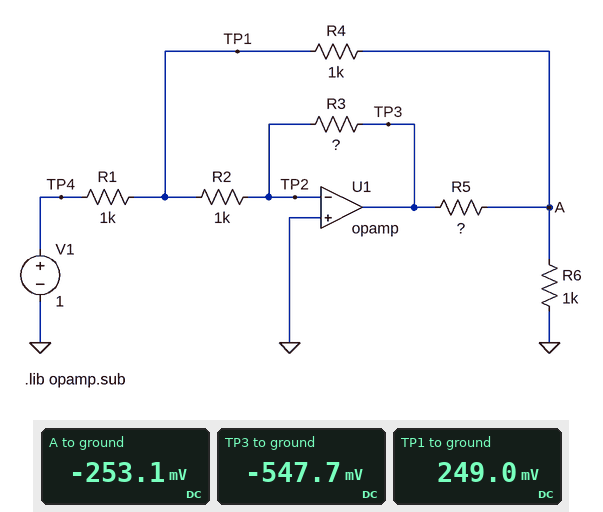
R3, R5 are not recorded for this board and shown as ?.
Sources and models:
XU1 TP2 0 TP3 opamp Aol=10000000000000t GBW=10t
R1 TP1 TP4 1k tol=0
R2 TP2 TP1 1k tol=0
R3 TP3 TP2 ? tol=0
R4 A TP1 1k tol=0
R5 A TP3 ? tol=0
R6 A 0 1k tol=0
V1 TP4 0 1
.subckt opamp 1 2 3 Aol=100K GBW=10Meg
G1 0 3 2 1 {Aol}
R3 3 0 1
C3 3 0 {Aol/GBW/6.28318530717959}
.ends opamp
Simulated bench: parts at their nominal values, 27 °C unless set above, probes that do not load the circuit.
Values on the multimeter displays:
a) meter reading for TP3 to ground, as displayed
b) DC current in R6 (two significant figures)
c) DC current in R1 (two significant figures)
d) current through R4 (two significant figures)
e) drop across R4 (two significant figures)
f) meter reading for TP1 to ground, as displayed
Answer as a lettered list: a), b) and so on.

a) -547.7 mV
b) 250 µA
c) 750 µA
d) 500 µA
e) 500 mV
f) 249.0 mV
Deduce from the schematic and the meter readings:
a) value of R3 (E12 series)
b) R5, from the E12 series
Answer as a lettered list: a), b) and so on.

a) 2.2 kΩ
b) 390 Ω
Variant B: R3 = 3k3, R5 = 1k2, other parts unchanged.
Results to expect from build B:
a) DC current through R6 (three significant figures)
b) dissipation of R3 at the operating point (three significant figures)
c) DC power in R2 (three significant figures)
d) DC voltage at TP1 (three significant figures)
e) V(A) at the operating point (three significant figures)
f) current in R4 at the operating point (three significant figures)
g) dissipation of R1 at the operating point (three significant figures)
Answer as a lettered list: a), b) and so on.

a) 171 µA
b) 252 µW
c) 76.4 µW
d) 276 mV
e) -171 mV
f) 447 µA
g) 524 µW
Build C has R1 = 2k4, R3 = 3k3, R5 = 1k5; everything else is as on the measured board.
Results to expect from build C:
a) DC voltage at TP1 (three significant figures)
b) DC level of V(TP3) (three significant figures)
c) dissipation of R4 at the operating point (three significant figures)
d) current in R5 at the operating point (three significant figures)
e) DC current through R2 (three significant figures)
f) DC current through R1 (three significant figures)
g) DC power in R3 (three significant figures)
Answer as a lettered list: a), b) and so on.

a) 145 mV
b) -480 mV
c) 44.4 µW
d) 276 µA
e) 145 µA
f) 356 µA
g) 69.7 µW
